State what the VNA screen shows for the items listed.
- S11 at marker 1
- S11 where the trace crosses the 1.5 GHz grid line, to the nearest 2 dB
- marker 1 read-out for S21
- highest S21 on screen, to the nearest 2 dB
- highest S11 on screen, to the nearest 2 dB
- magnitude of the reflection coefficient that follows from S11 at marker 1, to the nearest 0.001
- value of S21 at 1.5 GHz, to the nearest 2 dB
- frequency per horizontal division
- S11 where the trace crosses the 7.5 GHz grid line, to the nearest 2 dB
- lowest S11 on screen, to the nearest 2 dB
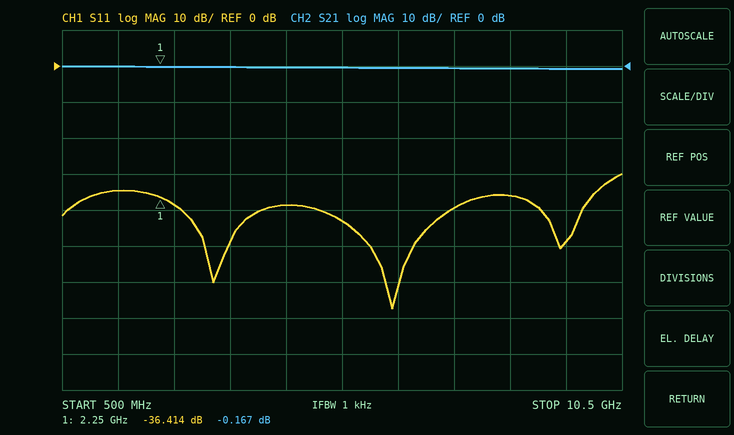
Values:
-36.414 dB
-34 dB
-0.167 dB
0 dB
-30 dB
0.015
0 dB
1 GHz
-40 dB
-68 dB
